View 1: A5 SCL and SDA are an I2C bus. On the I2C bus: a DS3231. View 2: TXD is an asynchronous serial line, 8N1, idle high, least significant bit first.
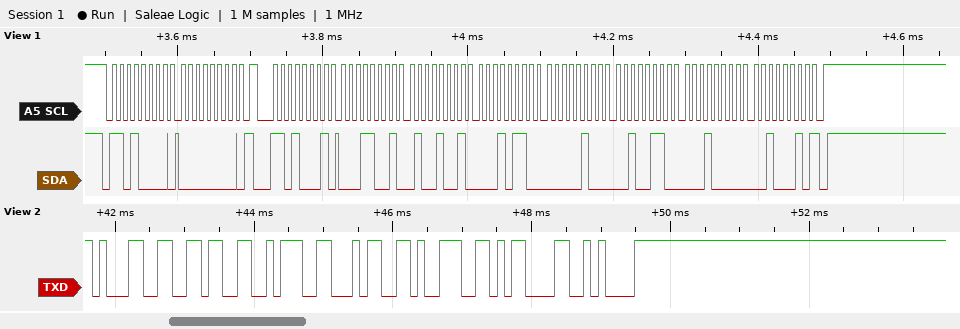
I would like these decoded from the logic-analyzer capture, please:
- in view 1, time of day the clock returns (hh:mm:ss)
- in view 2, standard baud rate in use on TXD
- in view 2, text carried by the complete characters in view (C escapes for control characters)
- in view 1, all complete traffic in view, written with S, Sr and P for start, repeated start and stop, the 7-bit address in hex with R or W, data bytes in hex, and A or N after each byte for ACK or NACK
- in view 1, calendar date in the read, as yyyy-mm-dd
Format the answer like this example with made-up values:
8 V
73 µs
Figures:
16:49:19
9600 baud
"16:49\r\n"
S 68W A 00 A Sr 68R A 19 A 49 A 16 A 04 A 26 A 10 A 22 N P
2022-10-26
